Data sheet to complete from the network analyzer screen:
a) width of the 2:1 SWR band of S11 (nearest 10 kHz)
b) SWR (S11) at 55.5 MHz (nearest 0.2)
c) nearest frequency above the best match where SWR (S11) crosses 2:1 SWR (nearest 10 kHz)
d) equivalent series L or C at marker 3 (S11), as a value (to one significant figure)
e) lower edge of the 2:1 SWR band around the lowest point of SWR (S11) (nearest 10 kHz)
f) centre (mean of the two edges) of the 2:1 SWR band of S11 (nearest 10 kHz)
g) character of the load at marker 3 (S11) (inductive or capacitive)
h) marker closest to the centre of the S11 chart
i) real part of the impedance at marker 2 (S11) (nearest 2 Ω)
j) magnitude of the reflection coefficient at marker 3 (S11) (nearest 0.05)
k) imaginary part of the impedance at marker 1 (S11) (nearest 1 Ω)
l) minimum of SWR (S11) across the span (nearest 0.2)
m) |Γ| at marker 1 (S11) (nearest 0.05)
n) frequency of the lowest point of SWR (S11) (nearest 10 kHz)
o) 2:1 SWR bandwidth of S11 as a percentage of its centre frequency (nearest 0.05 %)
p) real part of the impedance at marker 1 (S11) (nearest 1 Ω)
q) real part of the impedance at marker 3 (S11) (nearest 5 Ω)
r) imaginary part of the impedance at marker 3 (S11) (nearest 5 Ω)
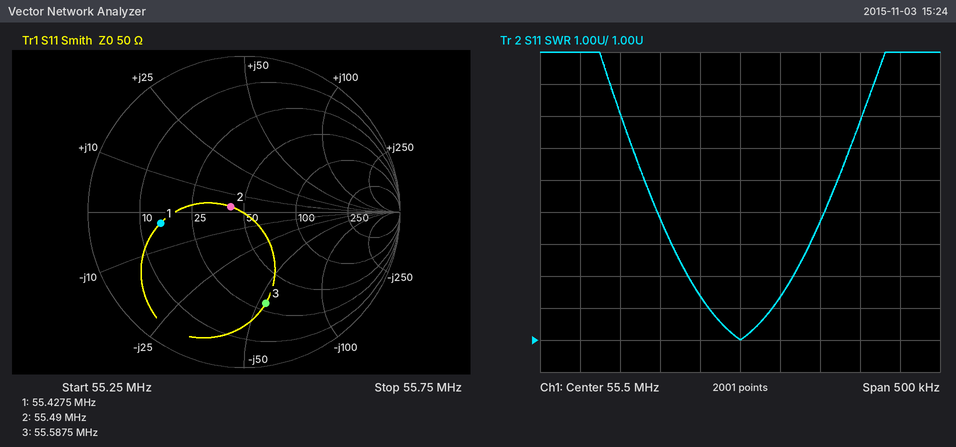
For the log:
80 kHz
1.0
55.54 MHz
50 pF
55.46 MHz
55.50 MHz
capacitive
marker 2
42 Ω
0.60
-3 Ω
1.0
0.55
55.50 MHz
0.15 %
15 Ω
30 Ω
-55 Ω
